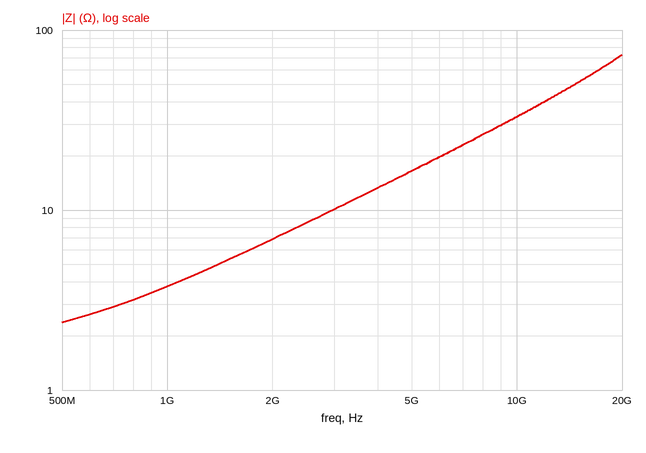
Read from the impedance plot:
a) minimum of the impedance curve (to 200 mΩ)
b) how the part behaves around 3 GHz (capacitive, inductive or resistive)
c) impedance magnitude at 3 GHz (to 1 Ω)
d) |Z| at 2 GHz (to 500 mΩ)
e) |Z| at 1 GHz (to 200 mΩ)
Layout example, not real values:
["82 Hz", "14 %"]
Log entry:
["2.4 Ω", "inductive", "10 Ω", "7.0 Ω", "3.8 Ω"]
